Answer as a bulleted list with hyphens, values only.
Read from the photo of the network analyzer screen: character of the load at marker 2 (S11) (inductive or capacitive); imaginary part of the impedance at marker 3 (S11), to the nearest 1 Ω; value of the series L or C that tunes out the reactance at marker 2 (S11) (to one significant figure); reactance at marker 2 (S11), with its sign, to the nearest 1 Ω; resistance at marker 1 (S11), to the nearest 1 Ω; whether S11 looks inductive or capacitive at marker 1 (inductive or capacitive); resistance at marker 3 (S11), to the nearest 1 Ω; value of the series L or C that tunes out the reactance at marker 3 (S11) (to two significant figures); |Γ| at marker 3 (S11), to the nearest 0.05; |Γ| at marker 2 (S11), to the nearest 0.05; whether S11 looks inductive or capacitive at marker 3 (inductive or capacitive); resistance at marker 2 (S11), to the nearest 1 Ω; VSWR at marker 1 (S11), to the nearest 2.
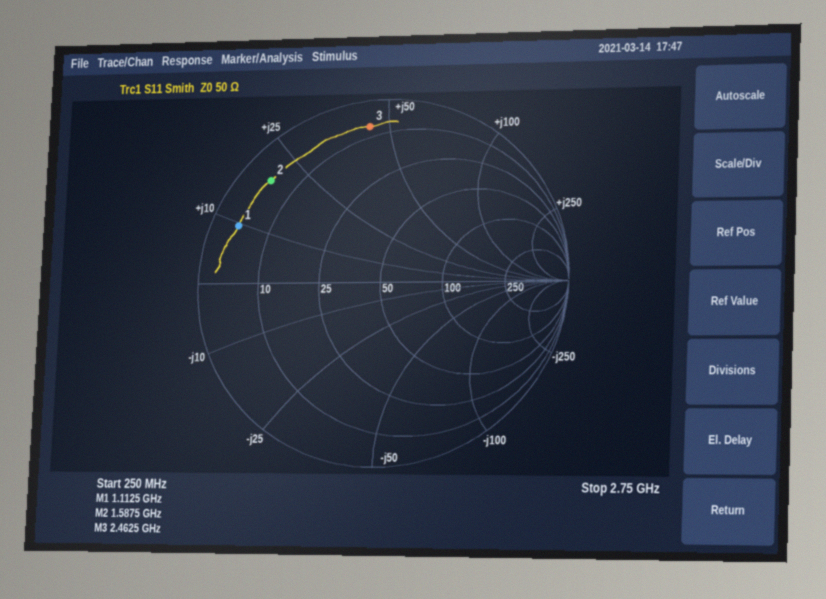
- inductive
- +44 Ω
- 5 pF
- +19 Ω
- 4 Ω
- inductive
- 7 Ω
- 1.5 pF
- 0.85
- 0.85
- inductive
- 5 Ω
- 12
